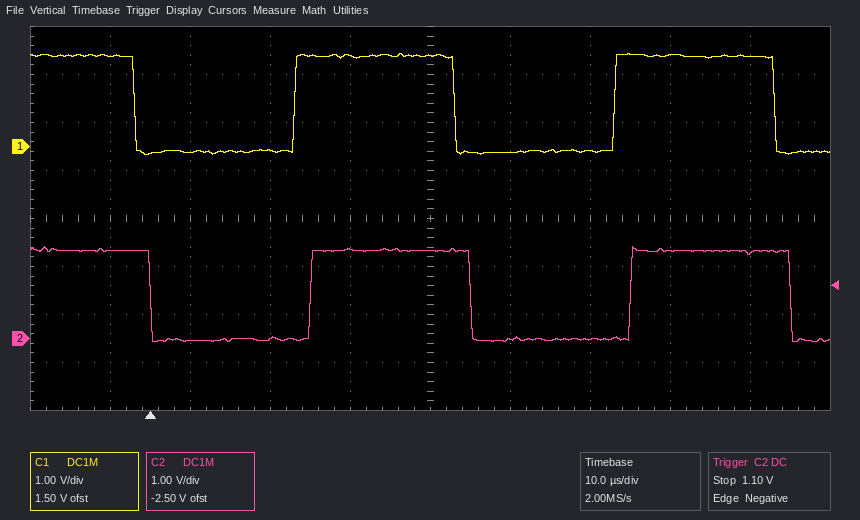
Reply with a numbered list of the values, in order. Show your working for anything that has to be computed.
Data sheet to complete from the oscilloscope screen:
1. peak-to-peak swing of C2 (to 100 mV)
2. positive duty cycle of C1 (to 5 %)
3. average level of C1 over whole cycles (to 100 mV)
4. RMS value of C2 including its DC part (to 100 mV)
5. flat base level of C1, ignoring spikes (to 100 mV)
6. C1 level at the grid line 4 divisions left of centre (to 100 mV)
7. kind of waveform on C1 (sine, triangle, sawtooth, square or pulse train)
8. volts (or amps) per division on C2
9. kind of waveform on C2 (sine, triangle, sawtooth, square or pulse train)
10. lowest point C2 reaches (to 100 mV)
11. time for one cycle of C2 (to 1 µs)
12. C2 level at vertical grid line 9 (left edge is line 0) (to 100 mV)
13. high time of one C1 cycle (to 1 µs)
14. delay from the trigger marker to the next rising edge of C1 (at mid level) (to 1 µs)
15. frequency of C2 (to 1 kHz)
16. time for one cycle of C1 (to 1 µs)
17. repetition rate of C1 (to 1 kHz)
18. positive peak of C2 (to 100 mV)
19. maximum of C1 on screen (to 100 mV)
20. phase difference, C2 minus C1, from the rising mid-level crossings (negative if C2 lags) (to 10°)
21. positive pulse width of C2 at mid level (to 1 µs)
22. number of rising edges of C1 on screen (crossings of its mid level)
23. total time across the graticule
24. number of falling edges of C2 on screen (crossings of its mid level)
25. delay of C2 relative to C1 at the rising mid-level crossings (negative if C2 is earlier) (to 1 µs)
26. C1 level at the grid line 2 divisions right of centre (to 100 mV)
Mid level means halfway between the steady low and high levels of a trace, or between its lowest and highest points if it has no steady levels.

1. 1.9 V − (-100 mV) = 2.0 V
2. 20 µs / 40 µs ≈ 50 %
3. -100 mV + 0.5 × (1.9 V − (-100 mV)) ≈ 900 mV
4. √(0.5 × (1.9 V)² + 0.5 × (-100 mV)²) ≈ 1.3 V
5. -100 mV
6. 1.9 V
7. square
8. 1 V
9. square
10. -100 mV
11. 40 µs
12. 1.8 V
13. 20 µs
14. 18 µs
15. 1 / 40 µs ≈ 25 kHz
16. 40 µs
17. 1 / 40 µs ≈ 25 kHz
18. 1.9 V
19. 1.9 V
20. −360° × (+2 µs) / 40 µs ≈ -18.0°, so -20° to the nearest 10°
21. 20 µs
22. 2
23. 100 µs
24. 3
25. +2 µs
26. -100 mV
